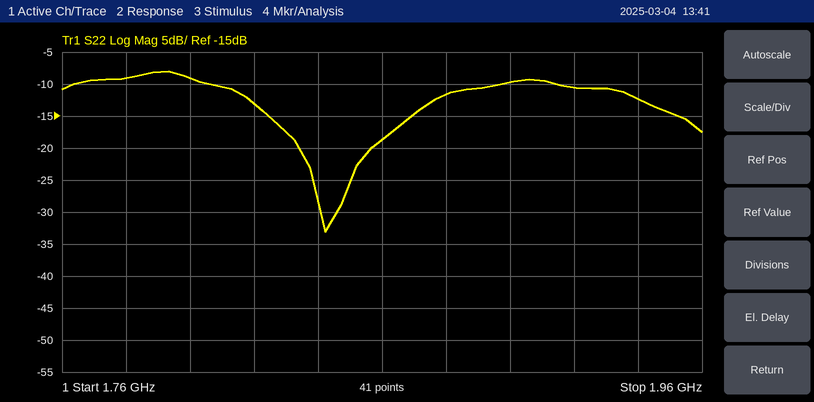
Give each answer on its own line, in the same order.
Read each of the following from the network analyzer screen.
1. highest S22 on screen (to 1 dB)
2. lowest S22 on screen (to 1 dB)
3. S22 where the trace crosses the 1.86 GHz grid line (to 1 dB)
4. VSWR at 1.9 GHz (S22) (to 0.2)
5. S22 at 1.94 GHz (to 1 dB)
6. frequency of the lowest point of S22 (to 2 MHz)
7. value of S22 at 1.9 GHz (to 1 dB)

-8 dB
-33 dB
-19 dB
2.0
-12 dB
1.842 GHz
-10 dB
